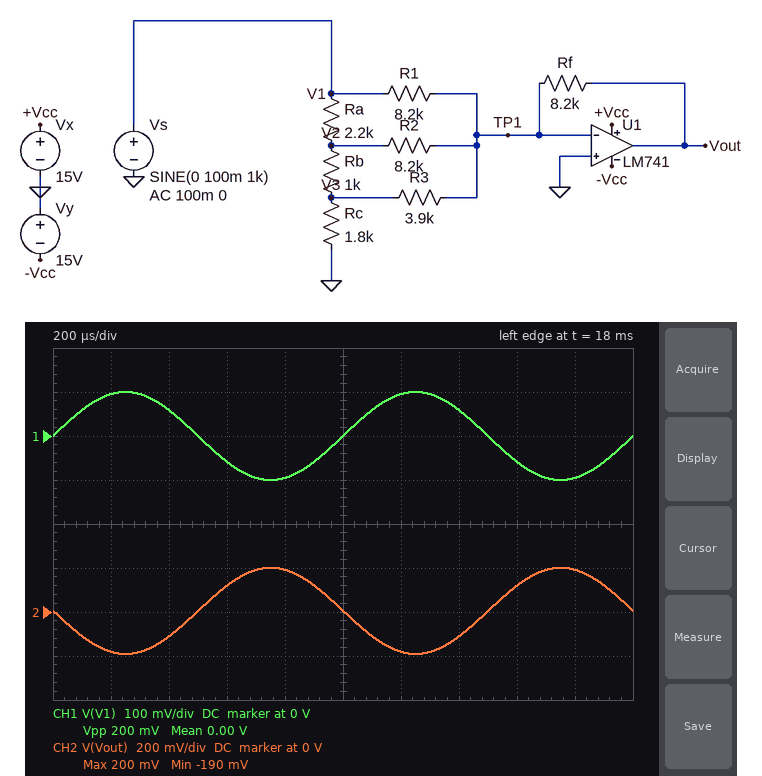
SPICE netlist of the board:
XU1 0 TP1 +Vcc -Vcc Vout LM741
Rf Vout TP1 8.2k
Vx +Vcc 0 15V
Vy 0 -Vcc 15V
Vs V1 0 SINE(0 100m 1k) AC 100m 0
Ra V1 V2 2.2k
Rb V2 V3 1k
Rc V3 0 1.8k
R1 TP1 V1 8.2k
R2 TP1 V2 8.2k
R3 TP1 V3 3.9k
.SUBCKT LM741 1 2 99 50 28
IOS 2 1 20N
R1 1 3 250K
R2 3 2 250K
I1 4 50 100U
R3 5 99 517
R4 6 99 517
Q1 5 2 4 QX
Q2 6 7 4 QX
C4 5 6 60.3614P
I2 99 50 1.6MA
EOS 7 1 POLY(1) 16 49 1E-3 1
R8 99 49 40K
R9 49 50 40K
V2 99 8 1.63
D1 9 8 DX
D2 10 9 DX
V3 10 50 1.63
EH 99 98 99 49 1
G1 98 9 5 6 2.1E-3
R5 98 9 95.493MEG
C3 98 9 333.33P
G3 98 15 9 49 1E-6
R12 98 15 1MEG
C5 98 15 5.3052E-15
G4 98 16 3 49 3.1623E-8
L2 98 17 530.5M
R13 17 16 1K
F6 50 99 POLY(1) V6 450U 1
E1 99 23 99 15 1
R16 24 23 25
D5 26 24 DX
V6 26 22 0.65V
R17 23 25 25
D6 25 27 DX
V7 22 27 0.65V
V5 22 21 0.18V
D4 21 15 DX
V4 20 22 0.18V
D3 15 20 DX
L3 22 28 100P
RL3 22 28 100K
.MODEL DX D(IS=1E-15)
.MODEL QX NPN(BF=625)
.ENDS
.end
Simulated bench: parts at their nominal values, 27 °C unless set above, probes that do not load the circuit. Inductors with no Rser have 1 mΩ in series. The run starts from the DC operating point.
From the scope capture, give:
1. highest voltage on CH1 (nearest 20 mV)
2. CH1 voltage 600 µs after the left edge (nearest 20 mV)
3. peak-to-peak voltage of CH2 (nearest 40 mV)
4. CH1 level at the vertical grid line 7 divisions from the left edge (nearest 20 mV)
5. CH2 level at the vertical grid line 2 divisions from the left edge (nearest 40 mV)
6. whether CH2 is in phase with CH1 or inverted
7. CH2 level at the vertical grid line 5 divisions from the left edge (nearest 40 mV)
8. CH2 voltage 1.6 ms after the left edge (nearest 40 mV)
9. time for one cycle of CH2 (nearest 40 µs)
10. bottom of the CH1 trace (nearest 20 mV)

100 mV
-60 mV
400 mV
60 mV
-120 mV
inverted
0 V
120 mV
1.00 ms
-100 mV
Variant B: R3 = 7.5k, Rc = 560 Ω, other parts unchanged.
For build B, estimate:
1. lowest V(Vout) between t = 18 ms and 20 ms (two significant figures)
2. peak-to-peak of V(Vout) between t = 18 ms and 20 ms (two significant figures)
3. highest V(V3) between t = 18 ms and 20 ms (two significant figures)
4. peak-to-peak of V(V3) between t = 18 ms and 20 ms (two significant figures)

-150 mV
300 mV
13 mV
25 mV
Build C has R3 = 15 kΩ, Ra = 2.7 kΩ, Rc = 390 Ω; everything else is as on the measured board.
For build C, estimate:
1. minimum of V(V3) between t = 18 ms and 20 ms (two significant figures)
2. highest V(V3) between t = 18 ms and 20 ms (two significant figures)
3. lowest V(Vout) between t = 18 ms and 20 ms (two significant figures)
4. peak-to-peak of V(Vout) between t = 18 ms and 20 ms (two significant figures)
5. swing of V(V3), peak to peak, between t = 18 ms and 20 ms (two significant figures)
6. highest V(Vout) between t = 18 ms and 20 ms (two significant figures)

-8.3 mV
8.4 mV
-130 mV
270 mV
17 mV
140 mV
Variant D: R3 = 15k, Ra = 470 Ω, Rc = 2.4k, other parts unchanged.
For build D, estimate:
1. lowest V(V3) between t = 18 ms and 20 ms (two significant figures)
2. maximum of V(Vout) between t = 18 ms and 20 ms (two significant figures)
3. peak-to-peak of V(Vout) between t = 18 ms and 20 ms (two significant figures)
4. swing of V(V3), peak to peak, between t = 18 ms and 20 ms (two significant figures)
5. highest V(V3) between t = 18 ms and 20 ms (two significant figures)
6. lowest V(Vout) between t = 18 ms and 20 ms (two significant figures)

-56 mV
220 mV
430 mV
110 mV
56 mV
-210 mV
